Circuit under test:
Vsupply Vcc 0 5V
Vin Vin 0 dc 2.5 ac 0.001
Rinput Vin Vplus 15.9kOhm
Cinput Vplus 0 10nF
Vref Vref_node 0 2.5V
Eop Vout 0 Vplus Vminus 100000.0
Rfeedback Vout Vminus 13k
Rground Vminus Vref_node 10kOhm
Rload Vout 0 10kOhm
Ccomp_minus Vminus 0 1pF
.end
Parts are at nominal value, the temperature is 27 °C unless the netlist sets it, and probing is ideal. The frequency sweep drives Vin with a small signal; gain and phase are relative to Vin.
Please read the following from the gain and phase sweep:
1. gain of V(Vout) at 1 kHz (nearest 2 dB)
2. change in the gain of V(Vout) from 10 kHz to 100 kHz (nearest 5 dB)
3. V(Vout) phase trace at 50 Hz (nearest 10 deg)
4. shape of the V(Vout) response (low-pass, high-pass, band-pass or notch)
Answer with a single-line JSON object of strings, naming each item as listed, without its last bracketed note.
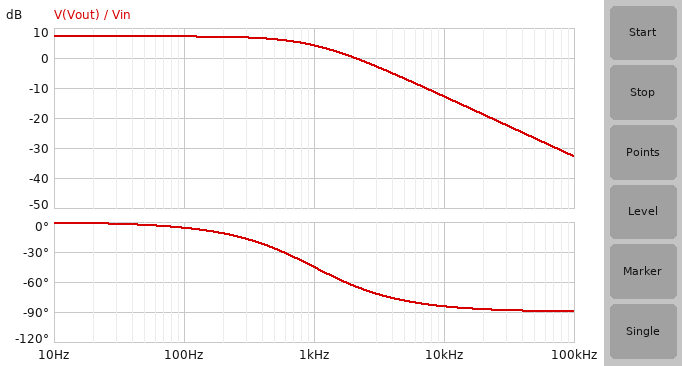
{"gain of V(Vout) at 1 kHz": "4 dB", "change in the gain of V(Vout) from 10 kHz to 100 kHz": "-20 dB", "V(Vout) phase trace at 50 Hz": "0 deg", "shape of the V(Vout) response": "low-pass"}
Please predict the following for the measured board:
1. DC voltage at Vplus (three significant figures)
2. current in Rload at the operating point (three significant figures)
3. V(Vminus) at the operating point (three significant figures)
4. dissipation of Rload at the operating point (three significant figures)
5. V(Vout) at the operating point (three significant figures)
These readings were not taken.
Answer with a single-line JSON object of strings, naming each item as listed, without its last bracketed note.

{"DC voltage at Vplus": "2.50 V", "current in Rload at the operating point": "250 µA", "V(Vminus) at the operating point": "2.50 V", "dissipation of Rload at the operating point": "625 µW", "V(Vout) at the operating point": "2.50 V"}
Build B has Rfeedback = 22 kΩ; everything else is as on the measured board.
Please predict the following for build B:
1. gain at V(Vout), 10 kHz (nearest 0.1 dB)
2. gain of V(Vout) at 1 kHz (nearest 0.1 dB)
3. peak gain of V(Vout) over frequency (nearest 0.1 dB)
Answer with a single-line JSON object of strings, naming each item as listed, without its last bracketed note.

{"gain at V(Vout), 10 kHz": "-9.9 dB", "gain of V(Vout) at 1 kHz": "7.1 dB", "peak gain of V(Vout) over frequency": "10.1 dB"}
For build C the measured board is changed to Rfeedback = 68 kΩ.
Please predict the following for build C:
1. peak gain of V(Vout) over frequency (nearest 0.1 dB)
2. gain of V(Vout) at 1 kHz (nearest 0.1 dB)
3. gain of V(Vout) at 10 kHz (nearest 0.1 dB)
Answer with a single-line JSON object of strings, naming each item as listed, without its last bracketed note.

{"peak gain of V(Vout) over frequency": "17.8 dB", "gain of V(Vout) at 1 kHz": "14.8 dB", "gain of V(Vout) at 10 kHz": "-2.2 dB"}
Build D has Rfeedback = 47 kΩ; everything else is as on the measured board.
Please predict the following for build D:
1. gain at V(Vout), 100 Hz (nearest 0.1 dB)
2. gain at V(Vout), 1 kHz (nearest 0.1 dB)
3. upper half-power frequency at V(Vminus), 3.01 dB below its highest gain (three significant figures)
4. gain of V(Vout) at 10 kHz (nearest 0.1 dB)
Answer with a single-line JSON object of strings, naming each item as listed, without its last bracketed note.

{"gain at V(Vout), 100 Hz": "15.1 dB", "gain at V(Vout), 1 kHz": "12.1 dB", "upper half-power frequency at V(Vminus), 3.01 dB below its highest gain": "1.00 kHz", "gain of V(Vout) at 10 kHz": "-4.9 dB"}
